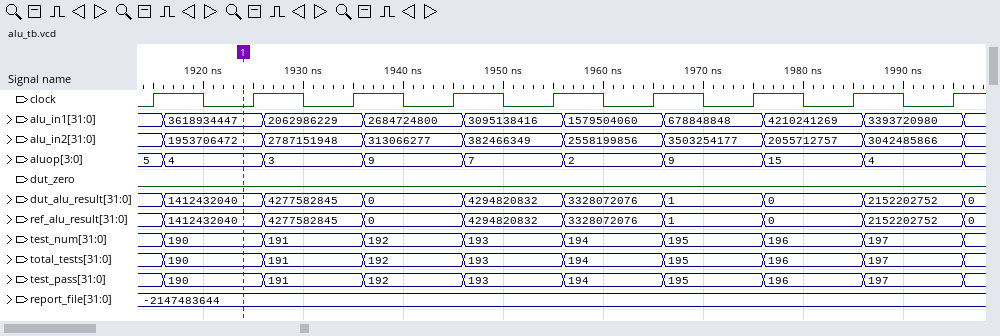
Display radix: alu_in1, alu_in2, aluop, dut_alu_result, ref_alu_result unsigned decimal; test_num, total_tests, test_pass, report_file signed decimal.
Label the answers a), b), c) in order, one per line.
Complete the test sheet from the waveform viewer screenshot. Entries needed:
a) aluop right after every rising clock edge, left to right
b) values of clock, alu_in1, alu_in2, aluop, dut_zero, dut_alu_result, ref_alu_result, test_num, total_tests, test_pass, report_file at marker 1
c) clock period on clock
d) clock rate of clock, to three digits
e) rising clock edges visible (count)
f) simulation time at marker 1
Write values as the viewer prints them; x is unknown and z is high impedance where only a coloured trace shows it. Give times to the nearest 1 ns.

a) 5, 4, 3, 9, 7, 2, 9, 15, 4
b) clock=0, alu_in1=3618934447, alu_in2=1953706472, aluop=4, dut_zero=0, dut_alu_result=1412432040, ref_alu_result=1412432040, test_num=190, total_tests=190, test_pass=190, report_file=-2147483644
c) 10 ns
d) 100 MHz
e) 9
f) 1924 ns
